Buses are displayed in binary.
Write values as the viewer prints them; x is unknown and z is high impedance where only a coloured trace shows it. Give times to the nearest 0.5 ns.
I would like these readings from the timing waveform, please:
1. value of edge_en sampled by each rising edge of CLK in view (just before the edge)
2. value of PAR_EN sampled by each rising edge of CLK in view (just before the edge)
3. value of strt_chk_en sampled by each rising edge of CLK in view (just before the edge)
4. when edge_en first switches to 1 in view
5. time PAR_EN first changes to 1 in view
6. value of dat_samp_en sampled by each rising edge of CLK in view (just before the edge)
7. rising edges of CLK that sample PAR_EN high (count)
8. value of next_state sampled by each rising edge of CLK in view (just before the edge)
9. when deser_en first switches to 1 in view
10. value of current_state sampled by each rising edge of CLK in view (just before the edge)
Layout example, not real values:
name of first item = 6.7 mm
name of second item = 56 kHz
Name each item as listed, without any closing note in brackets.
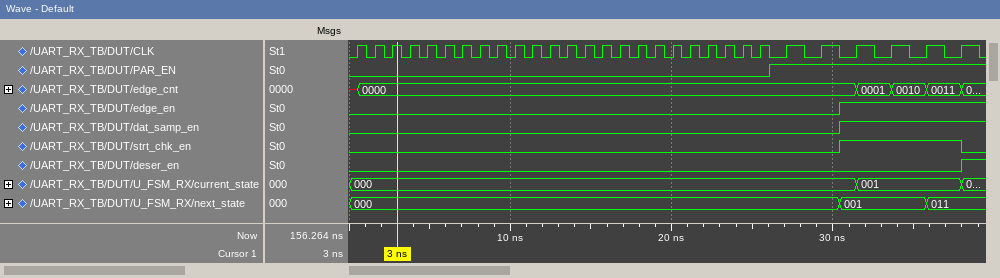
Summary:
value of edge_en sampled by each rising edge of CLK in view = 0 0 0 0 0 0 0 0 0 0 0 0 0 0 0 0 0 0 0 0 0 0 0 0 0 0 1 1 1 1
value of PAR_EN sampled by each rising edge of CLK in view = 0 0 0 0 0 0 0 0 0 0 0 0 0 0 0 0 0 0 0 0 0 0 0 0 1 1 1 1 1 1
value of strt_chk_en sampled by each rising edge of CLK in view = 0 0 0 0 0 0 0 0 0 0 0 0 0 0 0 0 0 0 0 0 0 0 0 0 0 0 1 1 1 1
when edge_en first switches to 1 in view = 30.5 ns
time PAR_EN first changes to 1 in view = 26 ns
value of dat_samp_en sampled by each rising edge of CLK in view = 0 0 0 0 0 0 0 0 0 0 0 0 0 0 0 0 0 0 0 0 0 0 0 0 0 0 1 1 1 1
rising edges of CLK that sample PAR_EN high = 6
value of next_state sampled by each rising edge of CLK in view = 000, 000, 000, 000, 000, 000, 000, 000, 000, 000, 000, 000, 000, 000, 000, 000, 000, 000, 000, 000, 000, 000, 000, 000, 000, 000, 001, 001, 001, 011
when deser_en first switches to 1 in view = 38 ns
value of current_state sampled by each rising edge of CLK in view = 000, 000, 000, 000, 000, 000, 000, 000, 000, 000, 000, 000, 000, 000, 000, 000, 000, 000, 000, 000, 000, 000, 000, 000, 000, 000, 000, 001, 001, 001
